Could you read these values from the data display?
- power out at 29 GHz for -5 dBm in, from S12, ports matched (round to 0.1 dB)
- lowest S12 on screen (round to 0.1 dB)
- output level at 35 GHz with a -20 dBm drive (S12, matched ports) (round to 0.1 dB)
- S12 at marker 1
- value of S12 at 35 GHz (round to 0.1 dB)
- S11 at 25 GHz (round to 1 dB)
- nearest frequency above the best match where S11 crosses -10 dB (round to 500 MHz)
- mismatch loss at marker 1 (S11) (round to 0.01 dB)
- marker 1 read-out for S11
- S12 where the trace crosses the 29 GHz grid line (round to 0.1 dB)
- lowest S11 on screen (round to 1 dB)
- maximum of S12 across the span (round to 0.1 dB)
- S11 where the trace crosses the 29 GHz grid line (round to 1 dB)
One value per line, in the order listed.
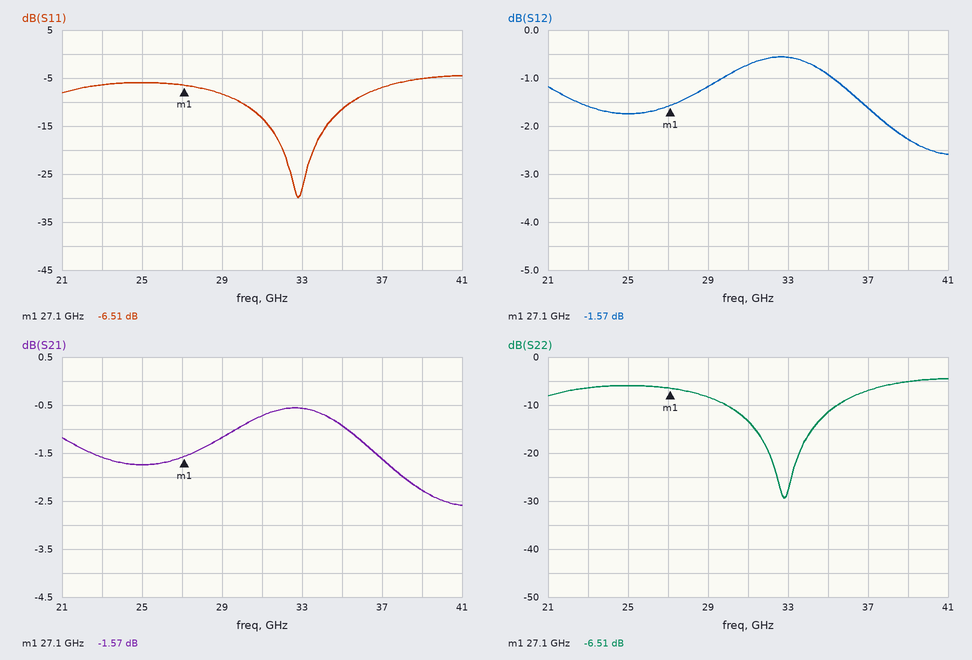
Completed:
-6.2 dBm
-2.6 dB
-20.9 dBm
-1.57 dB
-0.9 dB
-6 dB
35.5 GHz
1.10 dB
-6.51 dB
-1.2 dB
-30 dB
-0.6 dB
-8 dB
